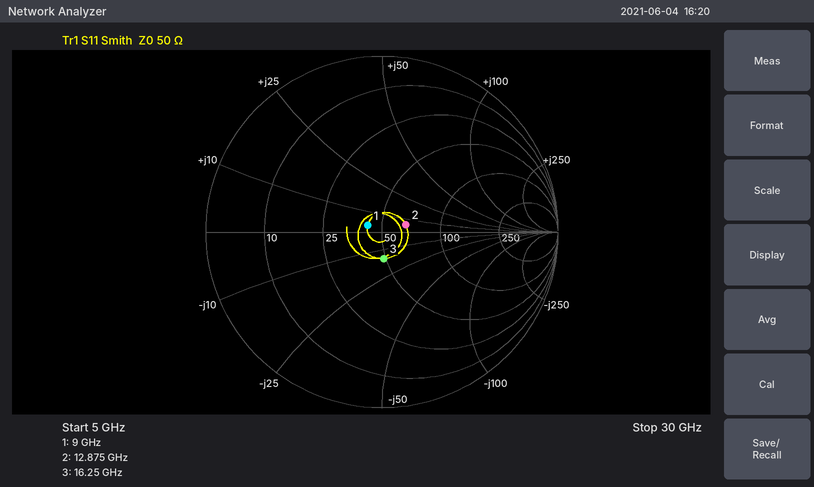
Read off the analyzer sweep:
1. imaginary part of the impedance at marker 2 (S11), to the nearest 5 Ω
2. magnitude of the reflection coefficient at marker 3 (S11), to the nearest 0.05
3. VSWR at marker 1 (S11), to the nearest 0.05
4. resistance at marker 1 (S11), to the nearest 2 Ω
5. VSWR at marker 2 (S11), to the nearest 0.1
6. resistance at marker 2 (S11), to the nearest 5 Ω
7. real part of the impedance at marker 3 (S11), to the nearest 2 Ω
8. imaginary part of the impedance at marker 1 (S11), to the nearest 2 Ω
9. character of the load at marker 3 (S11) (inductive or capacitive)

+5 Ω
0.15
1.20
42 Ω
1.3
65 Ω
48 Ω
+4 Ω
capacitive
